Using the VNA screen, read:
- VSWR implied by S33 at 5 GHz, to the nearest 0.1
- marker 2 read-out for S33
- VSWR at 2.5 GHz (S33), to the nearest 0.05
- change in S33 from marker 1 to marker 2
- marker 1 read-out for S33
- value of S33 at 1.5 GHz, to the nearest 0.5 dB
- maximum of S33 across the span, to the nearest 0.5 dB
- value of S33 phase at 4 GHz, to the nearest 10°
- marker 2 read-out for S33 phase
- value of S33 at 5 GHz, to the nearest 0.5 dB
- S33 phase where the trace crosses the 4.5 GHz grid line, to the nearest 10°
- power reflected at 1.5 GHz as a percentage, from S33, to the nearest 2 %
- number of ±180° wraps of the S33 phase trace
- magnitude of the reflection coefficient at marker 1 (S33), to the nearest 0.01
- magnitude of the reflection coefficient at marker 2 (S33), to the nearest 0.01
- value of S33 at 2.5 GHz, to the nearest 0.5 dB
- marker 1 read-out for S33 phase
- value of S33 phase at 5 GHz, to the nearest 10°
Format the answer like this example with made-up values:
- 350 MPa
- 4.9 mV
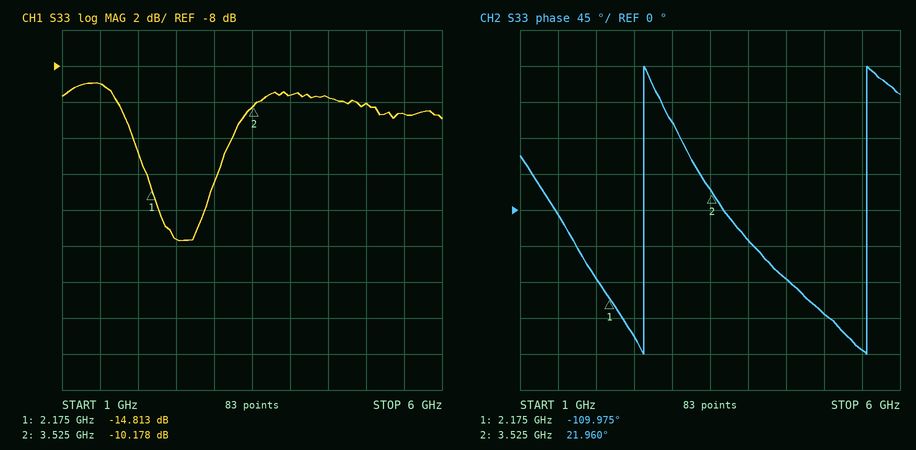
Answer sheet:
- 1.9
- -10.178 dB
- 1.30
- 4.635 dB
- -14.813 dB
- -9.0 dB
- -9.0 dB
- -40°
- 21.960°
- -10.0 dB
- -90°
- 12 %
- 2
- 0.18
- 0.31
- -17.5 dB
- -109.975°
- -130°
